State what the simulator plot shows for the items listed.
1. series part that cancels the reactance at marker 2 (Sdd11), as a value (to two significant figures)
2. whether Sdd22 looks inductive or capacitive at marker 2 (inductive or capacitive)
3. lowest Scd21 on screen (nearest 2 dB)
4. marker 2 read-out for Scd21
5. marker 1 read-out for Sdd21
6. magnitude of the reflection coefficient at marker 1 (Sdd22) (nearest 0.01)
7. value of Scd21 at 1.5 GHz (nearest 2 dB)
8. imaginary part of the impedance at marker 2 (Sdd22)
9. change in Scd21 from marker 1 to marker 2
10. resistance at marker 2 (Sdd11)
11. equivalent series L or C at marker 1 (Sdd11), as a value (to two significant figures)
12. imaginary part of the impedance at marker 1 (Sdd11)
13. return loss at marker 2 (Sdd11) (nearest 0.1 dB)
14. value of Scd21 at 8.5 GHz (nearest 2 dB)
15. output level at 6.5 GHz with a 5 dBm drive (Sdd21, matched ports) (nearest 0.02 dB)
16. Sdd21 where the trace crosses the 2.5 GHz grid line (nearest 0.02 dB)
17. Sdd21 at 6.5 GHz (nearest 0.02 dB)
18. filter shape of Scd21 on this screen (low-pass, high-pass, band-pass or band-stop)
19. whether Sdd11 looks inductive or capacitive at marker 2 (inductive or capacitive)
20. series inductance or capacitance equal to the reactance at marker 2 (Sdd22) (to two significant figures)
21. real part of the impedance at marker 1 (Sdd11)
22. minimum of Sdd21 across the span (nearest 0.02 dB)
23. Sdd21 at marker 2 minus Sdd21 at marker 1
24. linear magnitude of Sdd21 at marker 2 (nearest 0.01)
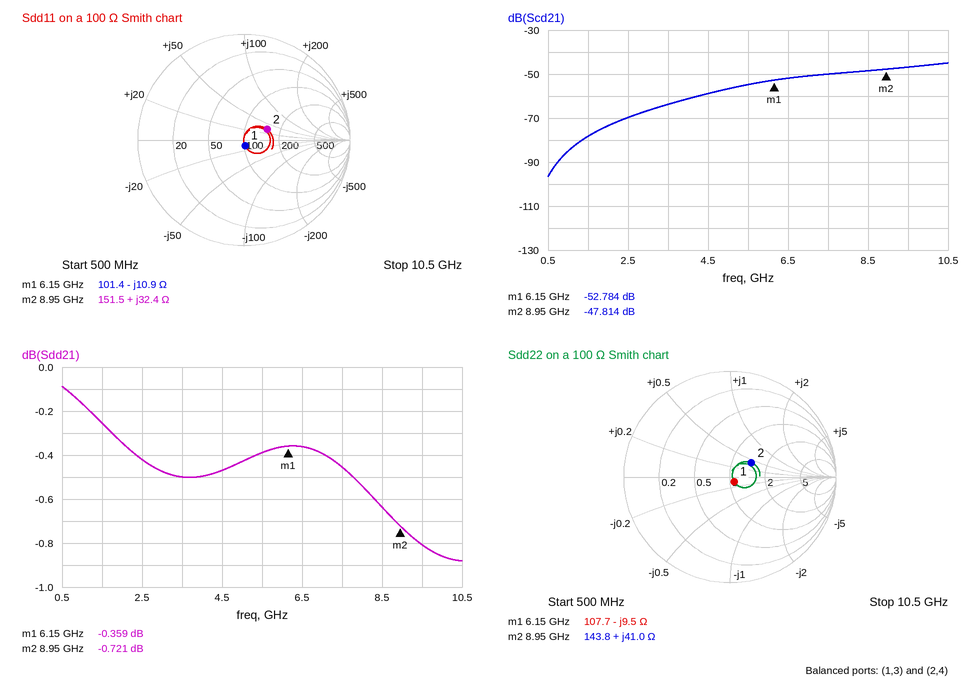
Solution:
550 fF
inductive
-96 dB
-47.814 dB
-0.359 dB
0.06
-78 dB
+41.0 Ω
4.970 dB
151.5 Ω
2.4 pF
-10.9 Ω
12.4 dB
-48 dB
4.64 dBm
-0.42 dB
-0.36 dB
high-pass
inductive
730 pH
101.4 Ω
-0.88 dB
-0.362 dB
0.92
